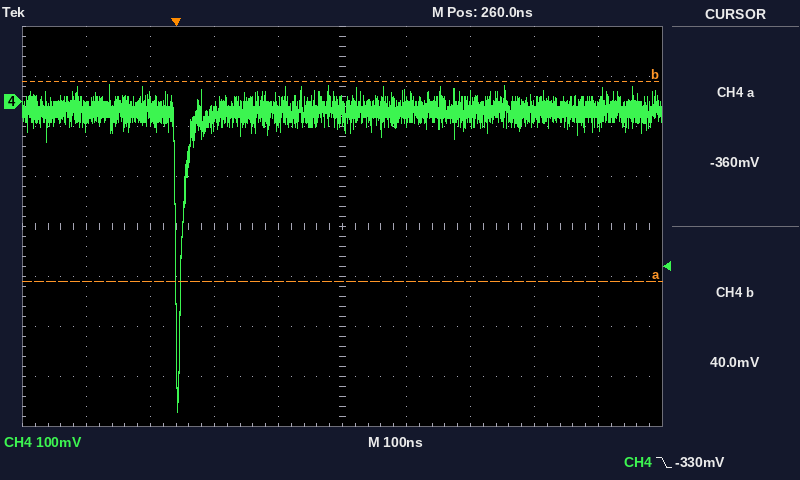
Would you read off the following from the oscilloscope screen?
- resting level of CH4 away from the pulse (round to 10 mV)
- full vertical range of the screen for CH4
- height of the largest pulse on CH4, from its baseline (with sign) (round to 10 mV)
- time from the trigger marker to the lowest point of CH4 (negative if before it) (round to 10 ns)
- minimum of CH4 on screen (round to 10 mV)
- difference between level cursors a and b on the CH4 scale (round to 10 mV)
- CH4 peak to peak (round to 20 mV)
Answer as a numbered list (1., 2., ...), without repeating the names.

1. -20 mV
2. 800 mV
3. -600 mV
4. 0 ns
5. -620 mV
6. 400 mV
7. 660 mV
